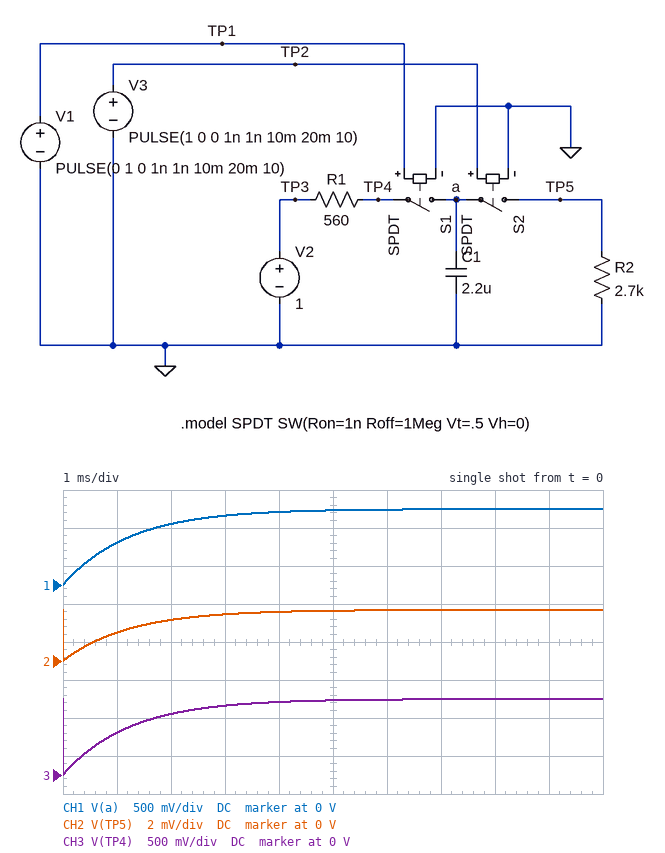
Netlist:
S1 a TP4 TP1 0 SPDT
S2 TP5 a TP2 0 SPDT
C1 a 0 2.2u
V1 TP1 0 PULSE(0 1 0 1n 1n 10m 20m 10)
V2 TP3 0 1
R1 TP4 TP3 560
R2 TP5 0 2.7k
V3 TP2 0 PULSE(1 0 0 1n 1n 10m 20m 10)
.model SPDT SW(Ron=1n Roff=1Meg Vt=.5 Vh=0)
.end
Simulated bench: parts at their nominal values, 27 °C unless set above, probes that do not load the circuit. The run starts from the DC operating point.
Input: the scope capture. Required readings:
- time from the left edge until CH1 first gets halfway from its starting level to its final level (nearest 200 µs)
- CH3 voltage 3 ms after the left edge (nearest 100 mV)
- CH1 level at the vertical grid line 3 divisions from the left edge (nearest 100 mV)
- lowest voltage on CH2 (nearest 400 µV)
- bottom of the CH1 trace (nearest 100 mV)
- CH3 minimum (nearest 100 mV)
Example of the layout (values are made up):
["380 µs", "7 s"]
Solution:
["800 µs", "900 mV", "900 mV", "0 V", "0 V", "0 V"]
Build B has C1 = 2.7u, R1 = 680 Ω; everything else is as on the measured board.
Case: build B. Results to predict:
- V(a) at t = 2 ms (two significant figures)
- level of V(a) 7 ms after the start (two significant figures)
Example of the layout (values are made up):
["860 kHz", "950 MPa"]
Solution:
["660 mV", "980 mV"]
